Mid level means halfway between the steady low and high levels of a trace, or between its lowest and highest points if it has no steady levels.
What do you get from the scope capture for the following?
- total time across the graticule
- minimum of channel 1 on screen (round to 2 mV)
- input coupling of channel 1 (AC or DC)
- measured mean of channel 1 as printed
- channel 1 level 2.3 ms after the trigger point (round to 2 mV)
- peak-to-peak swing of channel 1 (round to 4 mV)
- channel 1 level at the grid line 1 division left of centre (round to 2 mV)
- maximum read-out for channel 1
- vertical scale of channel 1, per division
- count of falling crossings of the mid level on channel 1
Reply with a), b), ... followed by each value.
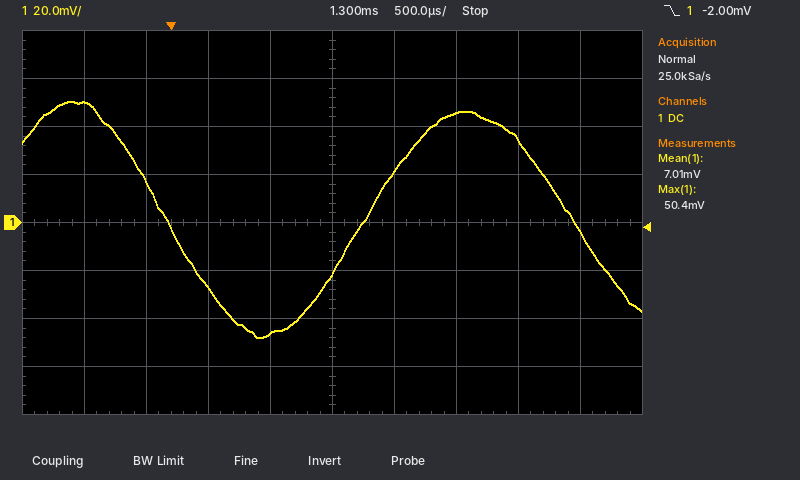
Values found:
a) 5 ms
b) -48 mV
c) DC
d) 7.01 mV
e) 46 mV
f) 100 mV
g) -46 mV
h) 50.4 mV
i) 20 mV
j) 2
